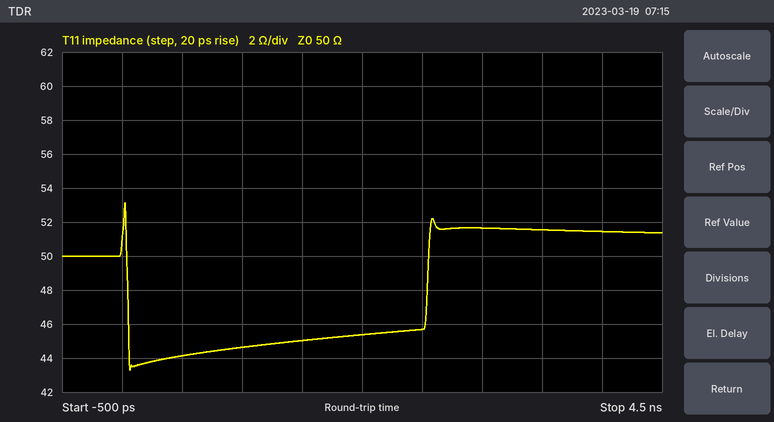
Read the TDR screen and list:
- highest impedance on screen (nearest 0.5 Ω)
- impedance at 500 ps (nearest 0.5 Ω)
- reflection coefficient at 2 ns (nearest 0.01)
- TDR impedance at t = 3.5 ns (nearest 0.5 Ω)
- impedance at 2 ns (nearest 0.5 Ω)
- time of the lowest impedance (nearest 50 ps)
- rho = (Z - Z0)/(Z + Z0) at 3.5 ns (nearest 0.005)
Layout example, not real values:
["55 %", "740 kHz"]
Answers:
["53.0 Ω", "44.0 Ω", "-0.05", "51.5 Ω", "45.5 Ω", "50 ps", "+0.015"]
